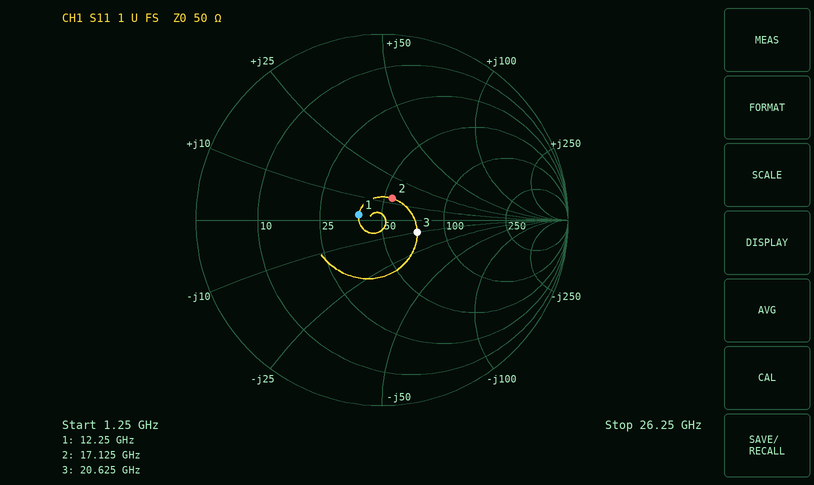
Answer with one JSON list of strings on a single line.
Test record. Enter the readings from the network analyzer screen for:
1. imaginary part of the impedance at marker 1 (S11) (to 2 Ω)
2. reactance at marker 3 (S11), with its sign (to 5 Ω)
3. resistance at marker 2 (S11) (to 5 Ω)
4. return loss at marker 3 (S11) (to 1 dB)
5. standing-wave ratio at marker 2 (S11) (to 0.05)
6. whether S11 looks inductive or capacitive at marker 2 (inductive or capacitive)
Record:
["+2 Ω", "-10 Ω", "55 Ω", "14 dB", "1.30", "inductive"]
